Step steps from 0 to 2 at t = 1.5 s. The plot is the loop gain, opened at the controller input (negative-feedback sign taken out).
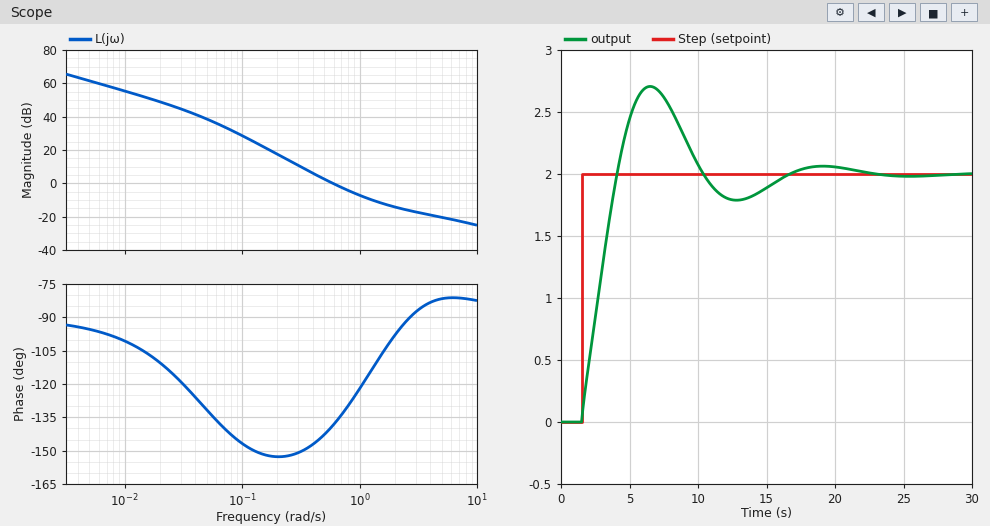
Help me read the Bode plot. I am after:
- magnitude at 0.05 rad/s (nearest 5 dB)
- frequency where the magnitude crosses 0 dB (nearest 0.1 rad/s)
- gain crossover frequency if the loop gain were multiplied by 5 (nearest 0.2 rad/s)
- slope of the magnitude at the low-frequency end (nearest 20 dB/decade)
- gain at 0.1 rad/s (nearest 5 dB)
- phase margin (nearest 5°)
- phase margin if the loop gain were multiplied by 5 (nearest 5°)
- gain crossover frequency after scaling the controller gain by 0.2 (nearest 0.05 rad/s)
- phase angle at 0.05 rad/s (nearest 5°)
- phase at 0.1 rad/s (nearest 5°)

40 dB
0.6 rad/s
2.0 rad/s
-20 dB/decade
30 dB
40°
80°
0.25 rad/s
-130°
-145°
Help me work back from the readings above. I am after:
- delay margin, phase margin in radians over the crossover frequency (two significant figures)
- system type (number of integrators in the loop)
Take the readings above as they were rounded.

1.2 s
1
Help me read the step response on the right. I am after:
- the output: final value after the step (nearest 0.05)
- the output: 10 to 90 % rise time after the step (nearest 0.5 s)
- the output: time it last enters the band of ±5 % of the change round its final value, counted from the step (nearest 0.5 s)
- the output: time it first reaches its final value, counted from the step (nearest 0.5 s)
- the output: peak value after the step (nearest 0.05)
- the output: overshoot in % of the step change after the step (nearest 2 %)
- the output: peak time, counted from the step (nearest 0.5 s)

2.00
2.0 s
13.5 s
2.5 s
2.70
36 %
5.0 s
